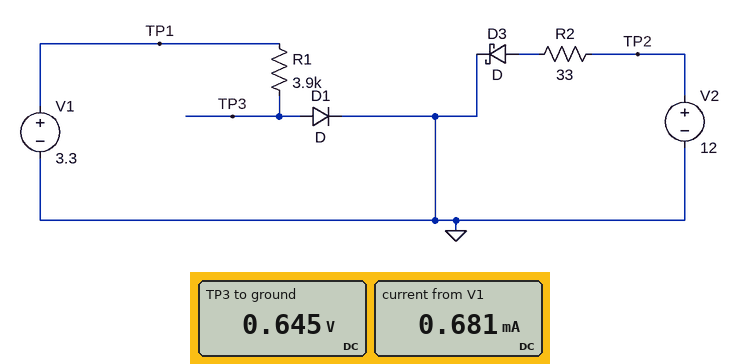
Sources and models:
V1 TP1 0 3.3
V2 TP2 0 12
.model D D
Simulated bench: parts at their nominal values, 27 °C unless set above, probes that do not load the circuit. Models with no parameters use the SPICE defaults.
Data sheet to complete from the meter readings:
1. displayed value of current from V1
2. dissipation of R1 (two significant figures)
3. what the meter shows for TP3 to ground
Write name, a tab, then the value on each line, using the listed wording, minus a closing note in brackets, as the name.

displayed value of current from V1	0.681 mA
dissipation of R1	1.8 mW
what the meter shows for TP3 to ground	0.645 V
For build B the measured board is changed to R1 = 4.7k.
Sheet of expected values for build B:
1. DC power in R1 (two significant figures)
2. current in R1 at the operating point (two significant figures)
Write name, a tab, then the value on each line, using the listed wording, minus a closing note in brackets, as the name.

DC power in R1	1.5 mW
current in R1 at the operating point	570 µA
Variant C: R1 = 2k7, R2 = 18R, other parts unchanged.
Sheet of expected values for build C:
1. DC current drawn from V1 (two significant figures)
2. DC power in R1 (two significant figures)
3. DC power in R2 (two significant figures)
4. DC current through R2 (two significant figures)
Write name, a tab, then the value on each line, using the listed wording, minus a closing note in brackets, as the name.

DC current drawn from V1	980 µA
DC power in R1	2.6 mW
DC power in R2	6.9 W
DC current through R2	620 mA
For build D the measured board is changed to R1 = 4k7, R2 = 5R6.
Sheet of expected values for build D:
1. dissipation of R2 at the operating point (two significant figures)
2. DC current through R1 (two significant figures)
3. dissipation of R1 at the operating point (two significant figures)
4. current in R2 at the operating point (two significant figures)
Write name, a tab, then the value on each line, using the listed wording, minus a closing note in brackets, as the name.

dissipation of R2 at the operating point	22 W
DC current through R1	570 µA
dissipation of R1 at the operating point	1.5 mW
current in R2 at the operating point	2.0 A
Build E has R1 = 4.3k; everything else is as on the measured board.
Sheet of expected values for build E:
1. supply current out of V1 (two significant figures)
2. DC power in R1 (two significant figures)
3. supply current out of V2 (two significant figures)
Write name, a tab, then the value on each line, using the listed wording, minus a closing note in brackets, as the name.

supply current out of V1	620 µA
DC power in R1	1.6 mW
supply current out of V2	340 mA
